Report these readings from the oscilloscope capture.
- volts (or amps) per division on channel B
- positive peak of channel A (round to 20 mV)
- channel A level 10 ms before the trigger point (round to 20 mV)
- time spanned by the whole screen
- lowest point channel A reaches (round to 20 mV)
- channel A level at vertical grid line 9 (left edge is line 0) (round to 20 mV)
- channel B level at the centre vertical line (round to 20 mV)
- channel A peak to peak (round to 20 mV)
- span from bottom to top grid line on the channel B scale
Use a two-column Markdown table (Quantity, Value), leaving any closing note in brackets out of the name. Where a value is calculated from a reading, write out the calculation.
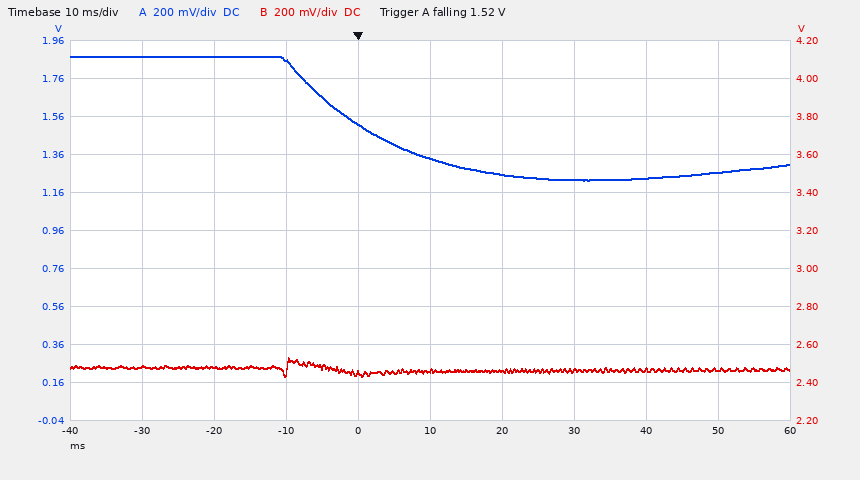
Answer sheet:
| Quantity | Value |
|---|---|
| volts (or amps) per division on channel B | 200 mV |
| positive peak of channel A | 1.88 V |
| channel A level 10 ms before the trigger point | 1.86 V |
| time spanned by the whole screen | 100 ms |
| lowest point channel A reaches | 1.22 V |
| channel A level at vertical grid line 9 (left edge is line 0) | 1.26 V |
| channel B level at the centre vertical line | 2.46 V |
| channel A peak to peak | 1.88 V − (1.22 V) = 660 mV |
| span from bottom to top grid line on the channel B scale | 2 V |
